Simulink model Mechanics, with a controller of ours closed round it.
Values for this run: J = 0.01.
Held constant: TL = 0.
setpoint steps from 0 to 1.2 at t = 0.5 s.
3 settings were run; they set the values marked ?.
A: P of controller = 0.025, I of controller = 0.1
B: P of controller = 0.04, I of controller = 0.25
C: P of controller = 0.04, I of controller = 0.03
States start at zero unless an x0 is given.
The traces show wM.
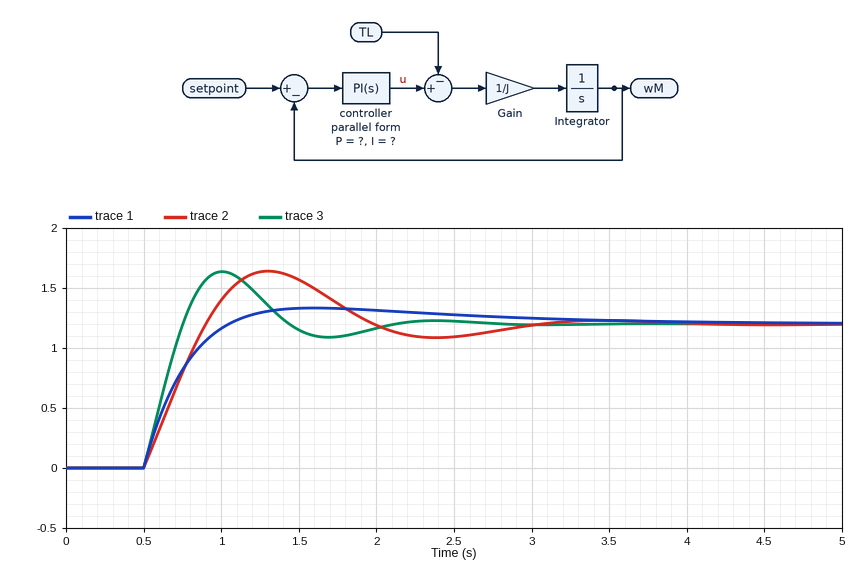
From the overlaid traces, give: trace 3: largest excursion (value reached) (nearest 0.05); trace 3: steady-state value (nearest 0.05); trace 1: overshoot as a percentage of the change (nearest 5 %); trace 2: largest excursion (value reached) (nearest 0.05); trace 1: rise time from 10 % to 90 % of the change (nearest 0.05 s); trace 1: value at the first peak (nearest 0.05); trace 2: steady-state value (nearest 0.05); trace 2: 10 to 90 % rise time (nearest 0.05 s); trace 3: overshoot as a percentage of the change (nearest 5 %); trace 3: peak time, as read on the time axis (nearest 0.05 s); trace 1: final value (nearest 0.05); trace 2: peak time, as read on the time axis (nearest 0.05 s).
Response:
1.65
1.20
10 %
1.65
0.40 s
1.35
1.20
0.30 s
35 %
1.00 s
1.20
1.30 s
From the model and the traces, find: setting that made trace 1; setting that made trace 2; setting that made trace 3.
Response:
C
A
B
